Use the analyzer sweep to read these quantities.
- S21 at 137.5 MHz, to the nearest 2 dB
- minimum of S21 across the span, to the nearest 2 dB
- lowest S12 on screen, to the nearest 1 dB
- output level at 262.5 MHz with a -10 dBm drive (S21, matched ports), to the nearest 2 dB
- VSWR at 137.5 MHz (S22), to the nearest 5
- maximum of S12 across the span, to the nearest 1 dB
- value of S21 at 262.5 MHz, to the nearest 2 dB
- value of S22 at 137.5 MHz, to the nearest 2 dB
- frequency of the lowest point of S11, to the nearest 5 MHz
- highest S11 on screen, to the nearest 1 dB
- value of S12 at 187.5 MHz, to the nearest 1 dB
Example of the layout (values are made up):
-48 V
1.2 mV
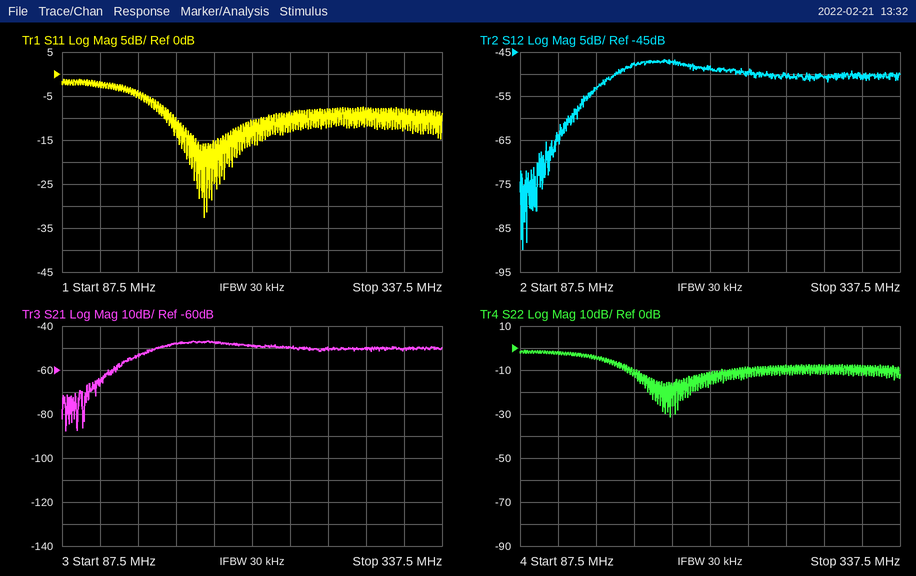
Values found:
-54 dB
-88 dB
-90 dB
-60 dBm
5
-47 dB
-50 dB
-4 dB
180 MHz
-1 dB
-47 dB
